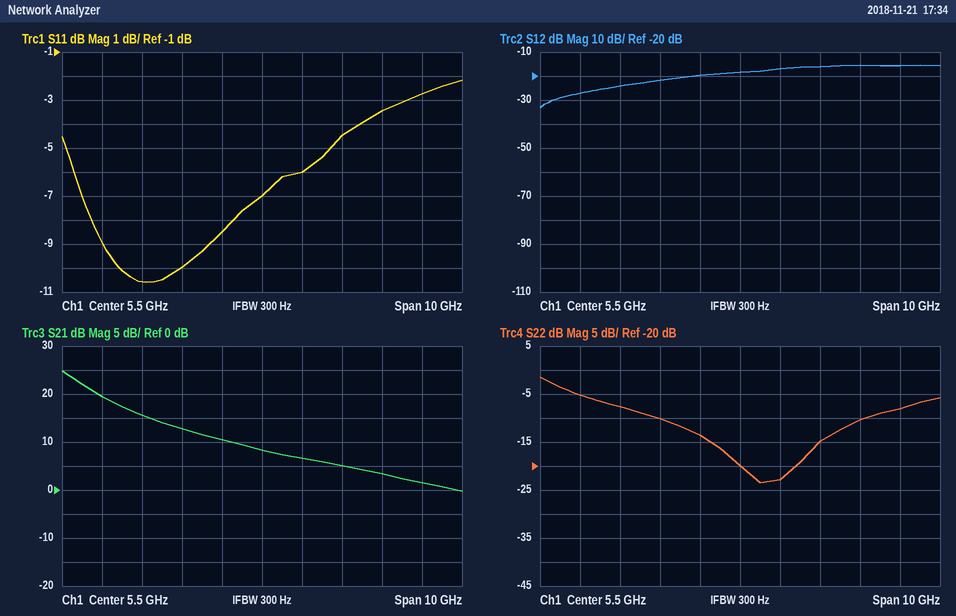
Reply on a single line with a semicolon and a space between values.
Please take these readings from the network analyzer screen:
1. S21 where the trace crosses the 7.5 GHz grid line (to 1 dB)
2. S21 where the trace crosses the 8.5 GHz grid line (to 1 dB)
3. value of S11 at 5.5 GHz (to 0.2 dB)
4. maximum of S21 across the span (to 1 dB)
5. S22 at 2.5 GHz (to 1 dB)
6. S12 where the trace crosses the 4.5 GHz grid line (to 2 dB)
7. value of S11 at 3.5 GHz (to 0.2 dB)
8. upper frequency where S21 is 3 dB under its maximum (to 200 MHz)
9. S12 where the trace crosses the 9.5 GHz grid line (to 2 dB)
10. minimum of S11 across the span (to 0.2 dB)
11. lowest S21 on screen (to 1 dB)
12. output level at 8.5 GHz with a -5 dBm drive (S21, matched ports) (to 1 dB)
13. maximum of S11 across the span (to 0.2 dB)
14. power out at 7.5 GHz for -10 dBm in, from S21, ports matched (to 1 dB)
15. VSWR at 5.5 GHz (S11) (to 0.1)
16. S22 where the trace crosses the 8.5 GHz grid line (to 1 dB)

5 dB; 3 dB; -7.0 dB; 25 dB; -8 dB; -20 dB; -10.0 dB; 1.0 GHz; -16 dB; -10.6 dB; 0 dB; -2 dBm; -2.2 dB; -5 dBm; 2.6; -10 dB
